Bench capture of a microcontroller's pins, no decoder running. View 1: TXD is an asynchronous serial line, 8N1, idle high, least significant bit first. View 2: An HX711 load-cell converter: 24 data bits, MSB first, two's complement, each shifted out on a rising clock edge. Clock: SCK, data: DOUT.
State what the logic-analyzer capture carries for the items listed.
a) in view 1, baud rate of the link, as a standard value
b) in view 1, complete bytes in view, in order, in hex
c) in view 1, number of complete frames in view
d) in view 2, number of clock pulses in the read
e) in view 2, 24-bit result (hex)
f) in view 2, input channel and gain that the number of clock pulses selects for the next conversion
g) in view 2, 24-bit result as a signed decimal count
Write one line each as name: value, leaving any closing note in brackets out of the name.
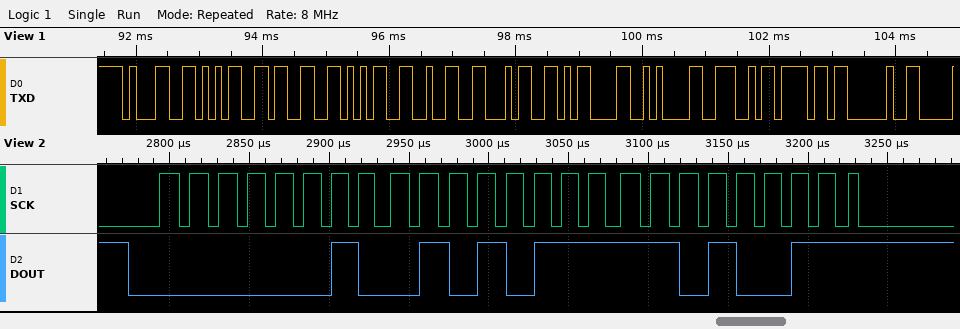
in view 1, baud rate of the link, as a standard value: 9600 baud
in view 1, complete bytes in view, in order, in hex: 31 35 33 35 32 34 0D 0A 4E 6F 20
in view 1, number of complete frames in view: 11
in view 2, number of clock pulses in the read: 25
in view 2, 24-bit result: 0x0257D3
in view 2, input channel and gain that the number of clock pulses selects for the next conversion: channel A, gain 128
in view 2, 24-bit result as a signed decimal count: 153555
